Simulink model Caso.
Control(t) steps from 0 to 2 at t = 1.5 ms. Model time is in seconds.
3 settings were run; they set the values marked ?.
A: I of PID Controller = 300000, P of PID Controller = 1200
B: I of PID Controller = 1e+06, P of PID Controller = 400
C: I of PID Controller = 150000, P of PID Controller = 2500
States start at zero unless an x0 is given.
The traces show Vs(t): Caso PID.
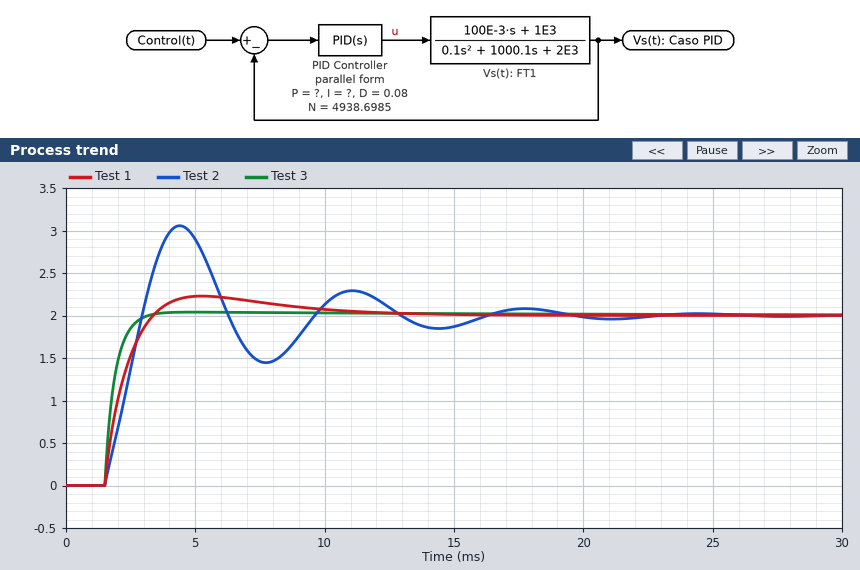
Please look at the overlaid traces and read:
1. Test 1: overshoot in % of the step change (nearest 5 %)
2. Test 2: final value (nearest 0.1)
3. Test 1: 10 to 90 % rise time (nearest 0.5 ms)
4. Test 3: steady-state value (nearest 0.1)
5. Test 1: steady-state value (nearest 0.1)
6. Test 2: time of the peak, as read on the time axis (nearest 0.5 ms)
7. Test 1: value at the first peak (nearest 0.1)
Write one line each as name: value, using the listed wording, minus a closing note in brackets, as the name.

Test 1: overshoot in % of the step change: 10 %
Test 2: final value: 2.0
Test 1: 10 to 90 % rise time: 1.5 ms
Test 3: steady-state value: 2.0
Test 1: steady-state value: 2.0
Test 2: time of the peak, as read on the time axis: 4.5 ms
Test 1: value at the first peak: 2.2
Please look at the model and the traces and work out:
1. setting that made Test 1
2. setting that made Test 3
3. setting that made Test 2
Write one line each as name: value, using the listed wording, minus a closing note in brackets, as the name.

setting that made Test 1: A
setting that made Test 3: C
setting that made Test 2: B
